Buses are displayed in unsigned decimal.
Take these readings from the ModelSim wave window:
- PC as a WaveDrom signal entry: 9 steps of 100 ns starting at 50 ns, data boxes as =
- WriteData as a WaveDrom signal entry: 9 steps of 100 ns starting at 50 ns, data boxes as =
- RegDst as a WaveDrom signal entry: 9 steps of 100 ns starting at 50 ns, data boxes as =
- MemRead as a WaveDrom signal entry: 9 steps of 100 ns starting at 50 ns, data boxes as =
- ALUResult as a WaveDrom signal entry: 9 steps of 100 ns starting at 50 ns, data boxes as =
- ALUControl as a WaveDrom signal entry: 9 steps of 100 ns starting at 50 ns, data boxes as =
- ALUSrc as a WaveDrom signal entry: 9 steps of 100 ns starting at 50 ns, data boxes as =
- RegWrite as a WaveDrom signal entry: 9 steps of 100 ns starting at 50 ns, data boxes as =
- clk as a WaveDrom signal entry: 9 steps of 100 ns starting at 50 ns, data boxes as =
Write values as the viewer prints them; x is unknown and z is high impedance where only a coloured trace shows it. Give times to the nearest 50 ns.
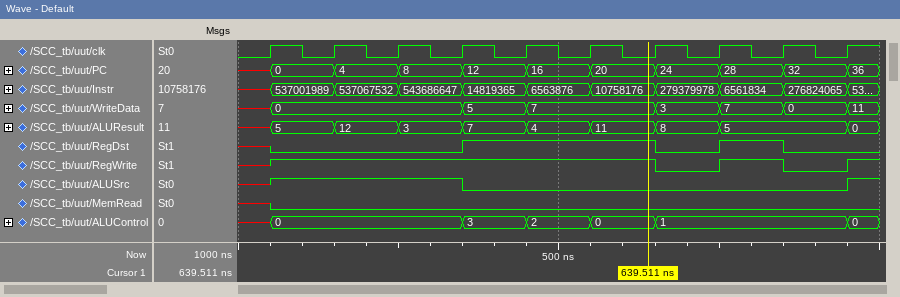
{name: 'PC', wave: '=========', data: '0 4 8 12 16 20 24 28 32'}
{name: 'WriteData', wave: '=..==.===', data: '0 5 7 3 7 0'}
{name: 'RegDst', wave: '0..1..010'}
{name: 'MemRead', wave: '0........'}
{name: 'ALUResult', wave: '========.', data: '5 12 3 7 4 11 8 5'}
{name: 'ALUControl', wave: '=..====..', data: '0 3 2 0 1'}
{name: 'ALUSrc', wave: '1..0.....'}
{name: 'RegWrite', wave: '1.....010'}
{name: 'clk', wave: 'p........'}
